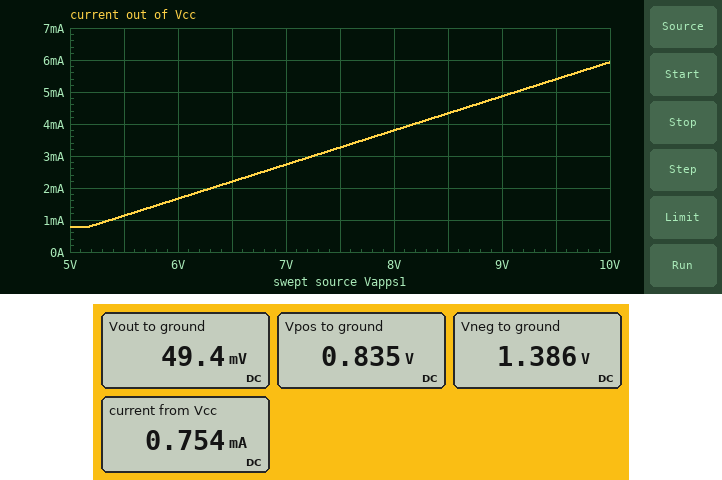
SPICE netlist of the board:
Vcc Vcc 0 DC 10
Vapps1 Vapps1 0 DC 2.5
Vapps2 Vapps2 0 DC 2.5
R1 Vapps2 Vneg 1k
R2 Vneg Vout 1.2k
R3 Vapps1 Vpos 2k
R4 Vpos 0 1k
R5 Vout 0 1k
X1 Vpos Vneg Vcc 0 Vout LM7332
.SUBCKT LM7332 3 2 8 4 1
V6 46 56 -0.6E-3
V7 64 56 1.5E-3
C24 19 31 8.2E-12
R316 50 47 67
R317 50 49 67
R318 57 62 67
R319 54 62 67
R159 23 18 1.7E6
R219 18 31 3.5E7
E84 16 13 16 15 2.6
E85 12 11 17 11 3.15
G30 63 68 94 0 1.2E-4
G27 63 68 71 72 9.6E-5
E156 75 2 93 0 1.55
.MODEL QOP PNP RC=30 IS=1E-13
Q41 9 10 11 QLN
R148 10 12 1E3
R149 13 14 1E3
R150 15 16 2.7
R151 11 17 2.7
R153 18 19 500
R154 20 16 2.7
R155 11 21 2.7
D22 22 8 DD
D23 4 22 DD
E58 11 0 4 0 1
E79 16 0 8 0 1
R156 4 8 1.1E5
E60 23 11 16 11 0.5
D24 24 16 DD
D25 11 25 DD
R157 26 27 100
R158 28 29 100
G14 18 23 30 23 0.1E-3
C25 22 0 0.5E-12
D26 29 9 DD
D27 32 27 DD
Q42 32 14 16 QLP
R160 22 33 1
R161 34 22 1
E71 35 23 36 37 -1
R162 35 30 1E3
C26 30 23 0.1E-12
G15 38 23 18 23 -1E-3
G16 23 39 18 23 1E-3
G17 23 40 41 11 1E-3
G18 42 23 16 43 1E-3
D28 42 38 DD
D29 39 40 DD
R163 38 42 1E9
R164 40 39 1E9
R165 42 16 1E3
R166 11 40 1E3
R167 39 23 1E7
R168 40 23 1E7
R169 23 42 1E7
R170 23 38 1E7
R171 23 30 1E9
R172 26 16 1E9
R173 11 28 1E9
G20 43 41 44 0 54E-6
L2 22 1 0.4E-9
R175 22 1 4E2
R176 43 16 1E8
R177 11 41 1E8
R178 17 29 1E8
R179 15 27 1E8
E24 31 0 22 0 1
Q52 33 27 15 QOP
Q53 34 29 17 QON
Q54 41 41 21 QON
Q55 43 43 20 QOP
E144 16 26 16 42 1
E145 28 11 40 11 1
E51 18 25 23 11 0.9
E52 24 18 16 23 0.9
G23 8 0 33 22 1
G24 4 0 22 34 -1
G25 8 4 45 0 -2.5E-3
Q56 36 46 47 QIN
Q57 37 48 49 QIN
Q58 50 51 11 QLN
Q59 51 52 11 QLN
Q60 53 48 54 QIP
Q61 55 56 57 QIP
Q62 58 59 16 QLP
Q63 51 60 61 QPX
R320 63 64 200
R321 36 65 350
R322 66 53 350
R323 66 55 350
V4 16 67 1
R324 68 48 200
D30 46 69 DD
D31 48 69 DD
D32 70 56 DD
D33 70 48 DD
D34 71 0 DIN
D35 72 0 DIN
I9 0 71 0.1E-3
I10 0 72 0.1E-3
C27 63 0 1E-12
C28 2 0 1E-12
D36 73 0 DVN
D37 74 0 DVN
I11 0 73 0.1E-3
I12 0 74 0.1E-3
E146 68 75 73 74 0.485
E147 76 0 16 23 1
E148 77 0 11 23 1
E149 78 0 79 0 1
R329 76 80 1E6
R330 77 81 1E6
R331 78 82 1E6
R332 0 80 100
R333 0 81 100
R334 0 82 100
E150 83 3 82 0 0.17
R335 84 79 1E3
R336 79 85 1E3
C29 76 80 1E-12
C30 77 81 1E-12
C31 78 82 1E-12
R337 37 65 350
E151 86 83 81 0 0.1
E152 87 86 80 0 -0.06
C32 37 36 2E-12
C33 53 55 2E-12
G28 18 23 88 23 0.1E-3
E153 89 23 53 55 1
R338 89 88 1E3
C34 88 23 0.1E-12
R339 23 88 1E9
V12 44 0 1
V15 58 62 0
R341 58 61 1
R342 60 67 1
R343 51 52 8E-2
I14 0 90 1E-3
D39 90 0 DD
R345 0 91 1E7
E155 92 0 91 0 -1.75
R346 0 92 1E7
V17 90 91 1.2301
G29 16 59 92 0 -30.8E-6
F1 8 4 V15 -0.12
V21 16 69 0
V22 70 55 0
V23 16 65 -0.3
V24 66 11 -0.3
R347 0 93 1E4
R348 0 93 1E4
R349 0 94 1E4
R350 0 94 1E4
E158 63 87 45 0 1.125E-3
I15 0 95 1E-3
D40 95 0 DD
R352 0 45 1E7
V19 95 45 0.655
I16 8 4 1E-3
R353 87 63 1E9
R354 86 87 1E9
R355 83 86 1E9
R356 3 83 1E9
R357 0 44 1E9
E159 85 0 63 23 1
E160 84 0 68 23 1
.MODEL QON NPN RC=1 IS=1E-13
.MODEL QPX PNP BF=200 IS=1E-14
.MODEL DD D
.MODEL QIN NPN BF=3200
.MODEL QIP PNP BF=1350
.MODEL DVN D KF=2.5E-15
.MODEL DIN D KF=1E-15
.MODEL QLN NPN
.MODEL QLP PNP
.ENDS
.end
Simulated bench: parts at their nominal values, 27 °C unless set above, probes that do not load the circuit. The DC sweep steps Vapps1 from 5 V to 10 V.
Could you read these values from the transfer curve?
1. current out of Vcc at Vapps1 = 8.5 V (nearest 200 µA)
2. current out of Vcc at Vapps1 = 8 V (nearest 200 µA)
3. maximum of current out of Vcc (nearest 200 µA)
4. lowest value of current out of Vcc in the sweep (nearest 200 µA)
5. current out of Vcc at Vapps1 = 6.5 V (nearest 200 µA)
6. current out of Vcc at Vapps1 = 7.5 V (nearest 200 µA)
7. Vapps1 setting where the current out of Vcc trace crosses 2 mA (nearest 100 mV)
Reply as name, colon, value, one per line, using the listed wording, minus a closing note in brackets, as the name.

current out of Vcc at Vapps1 = 8.5 V: 4.4 mA
current out of Vcc at Vapps1 = 8 V: 3.8 mA
maximum of current out of Vcc: 6.0 mA
lowest value of current out of Vcc in the sweep: 800 µA
current out of Vcc at Vapps1 = 6.5 V: 2.2 mA
current out of Vcc at Vapps1 = 7.5 V: 3.2 mA
Vapps1 setting where the current out of Vcc trace crosses 2 mA: 6.3 V
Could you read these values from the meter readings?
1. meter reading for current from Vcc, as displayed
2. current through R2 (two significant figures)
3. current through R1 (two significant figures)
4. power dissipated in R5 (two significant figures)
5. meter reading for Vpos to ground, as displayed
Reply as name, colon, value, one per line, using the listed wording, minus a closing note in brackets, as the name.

meter reading for current from Vcc, as displayed: 0.754 mA
current through R2: 1.1 mA
current through R1: 1.1 mA
power dissipated in R5: 2.4 µW
meter reading for Vpos to ground, as displayed: 0.835 V
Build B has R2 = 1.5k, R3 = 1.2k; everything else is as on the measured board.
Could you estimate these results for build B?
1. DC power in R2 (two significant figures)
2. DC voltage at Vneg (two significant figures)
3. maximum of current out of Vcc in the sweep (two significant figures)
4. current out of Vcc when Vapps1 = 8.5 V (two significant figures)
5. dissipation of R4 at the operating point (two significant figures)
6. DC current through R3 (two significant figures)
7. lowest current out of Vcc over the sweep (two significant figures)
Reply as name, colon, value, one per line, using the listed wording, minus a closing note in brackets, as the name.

DC power in R2: 1.4 mW
DC voltage at Vneg: 1.5 V
maximum of current out of Vcc in the sweep: 10 mA
current out of Vcc when Vapps1 = 8.5 V: 8.0 mA
dissipation of R4 at the operating point: 1.3 mW
DC current through R3: 1.1 mA
lowest current out of Vcc over the sweep: 2.5 mA
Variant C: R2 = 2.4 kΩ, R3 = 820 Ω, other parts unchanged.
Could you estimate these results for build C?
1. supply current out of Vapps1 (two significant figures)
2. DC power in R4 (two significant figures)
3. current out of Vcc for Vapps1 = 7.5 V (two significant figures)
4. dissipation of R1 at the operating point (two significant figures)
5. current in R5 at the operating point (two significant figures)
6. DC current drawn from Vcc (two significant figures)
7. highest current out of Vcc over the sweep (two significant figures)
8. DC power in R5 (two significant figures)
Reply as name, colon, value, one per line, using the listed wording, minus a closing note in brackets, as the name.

supply current out of Vapps1: 1.4 mA
DC power in R4: 1.9 mW
current out of Vcc for Vapps1 = 7.5 V: 10 mA
dissipation of R1 at the operating point: 520 µW
current in R5 at the operating point: 47 µA
DC current drawn from Vcc: 750 µA
highest current out of Vcc over the sweep: 12 mA
DC power in R5: 2.2 µW
